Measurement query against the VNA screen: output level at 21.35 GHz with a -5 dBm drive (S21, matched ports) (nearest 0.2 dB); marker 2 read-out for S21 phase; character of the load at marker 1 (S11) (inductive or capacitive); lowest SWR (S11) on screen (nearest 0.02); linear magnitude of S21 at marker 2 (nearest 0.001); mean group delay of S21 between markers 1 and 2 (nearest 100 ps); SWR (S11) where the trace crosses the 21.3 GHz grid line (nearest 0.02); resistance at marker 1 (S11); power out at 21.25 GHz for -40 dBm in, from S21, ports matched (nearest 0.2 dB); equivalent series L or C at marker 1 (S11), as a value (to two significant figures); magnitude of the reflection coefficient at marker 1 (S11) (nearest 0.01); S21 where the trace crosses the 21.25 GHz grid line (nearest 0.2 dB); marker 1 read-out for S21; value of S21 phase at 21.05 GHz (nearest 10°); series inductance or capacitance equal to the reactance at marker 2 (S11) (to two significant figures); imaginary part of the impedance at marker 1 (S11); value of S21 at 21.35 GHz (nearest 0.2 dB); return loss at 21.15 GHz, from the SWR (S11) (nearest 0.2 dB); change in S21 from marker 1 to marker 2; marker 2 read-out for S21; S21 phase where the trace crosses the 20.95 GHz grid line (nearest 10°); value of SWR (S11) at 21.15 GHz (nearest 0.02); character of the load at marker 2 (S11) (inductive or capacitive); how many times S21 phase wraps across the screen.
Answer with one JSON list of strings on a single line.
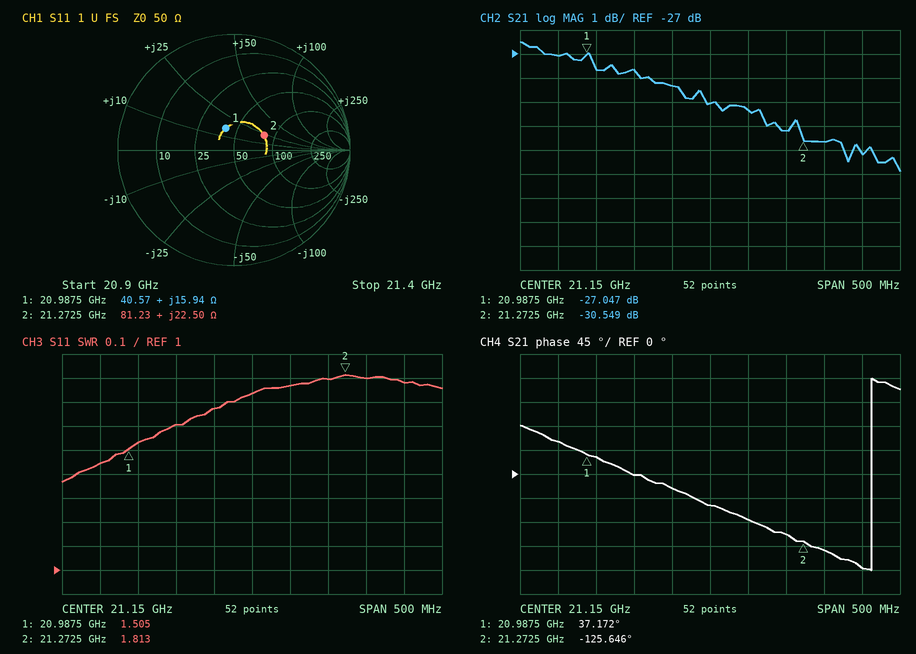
["-36.2 dBm", "-125.646°", "inductive", "1.36", "0.030", "1.6 ns", "1.80", "40.57 Ω", "-70.2 dBm", "120 pH", "0.20", "-30.2 dB", "-27.047 dB", "0°", "170 pH", "+15.94 Ω", "-31.2 dB", "11.4 dB", "-3.502 dB", "-30.549 dB", "60°", "1.74", "inductive", "1"]
